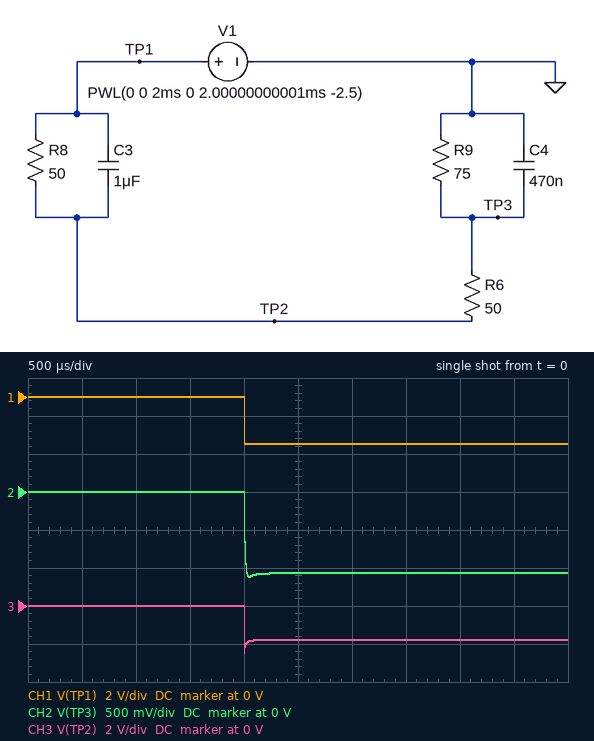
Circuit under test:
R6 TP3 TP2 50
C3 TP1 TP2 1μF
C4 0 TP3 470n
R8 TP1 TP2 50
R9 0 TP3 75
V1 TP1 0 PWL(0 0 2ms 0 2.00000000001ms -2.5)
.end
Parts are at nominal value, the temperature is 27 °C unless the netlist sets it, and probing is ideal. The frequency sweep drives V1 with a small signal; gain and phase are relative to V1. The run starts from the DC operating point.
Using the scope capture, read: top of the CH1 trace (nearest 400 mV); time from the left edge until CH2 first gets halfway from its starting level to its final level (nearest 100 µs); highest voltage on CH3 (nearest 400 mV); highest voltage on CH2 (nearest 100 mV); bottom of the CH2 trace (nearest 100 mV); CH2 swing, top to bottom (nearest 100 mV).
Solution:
0 V
2.0 ms
0 V
0 V
-1.1 V
1.1 V
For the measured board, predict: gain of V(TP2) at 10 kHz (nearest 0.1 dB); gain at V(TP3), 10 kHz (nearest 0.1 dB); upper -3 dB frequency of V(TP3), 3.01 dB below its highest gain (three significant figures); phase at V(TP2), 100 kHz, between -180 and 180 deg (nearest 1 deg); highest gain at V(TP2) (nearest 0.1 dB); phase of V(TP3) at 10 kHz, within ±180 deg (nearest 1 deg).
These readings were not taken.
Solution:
-1.3 dB
-8.2 dB
16.4 kHz
2 deg
0 dB
-33 deg
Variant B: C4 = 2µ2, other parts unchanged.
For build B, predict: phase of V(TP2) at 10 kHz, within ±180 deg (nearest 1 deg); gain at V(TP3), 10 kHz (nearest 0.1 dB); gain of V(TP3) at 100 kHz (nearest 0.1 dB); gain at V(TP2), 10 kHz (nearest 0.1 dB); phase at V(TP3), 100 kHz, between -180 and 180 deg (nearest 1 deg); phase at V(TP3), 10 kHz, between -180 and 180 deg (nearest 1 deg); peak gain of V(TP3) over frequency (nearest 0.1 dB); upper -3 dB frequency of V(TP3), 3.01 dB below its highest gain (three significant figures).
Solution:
13 deg
-18.3 dB
-36.8 dB
-1.3 dB
-87 deg
-63 deg
-7.4 dB
1.79 kHz
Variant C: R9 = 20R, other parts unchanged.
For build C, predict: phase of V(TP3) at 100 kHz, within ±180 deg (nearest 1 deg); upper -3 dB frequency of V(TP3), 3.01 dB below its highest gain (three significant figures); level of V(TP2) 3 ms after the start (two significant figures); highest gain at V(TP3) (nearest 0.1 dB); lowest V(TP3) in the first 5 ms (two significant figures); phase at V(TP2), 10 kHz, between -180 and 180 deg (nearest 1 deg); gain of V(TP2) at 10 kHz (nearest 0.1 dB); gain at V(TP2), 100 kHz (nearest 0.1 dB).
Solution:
-75 deg
31.8 kHz
-1.5 V
-12.6 dB
-560 mV
11 deg
-1.0 dB
0 dB
